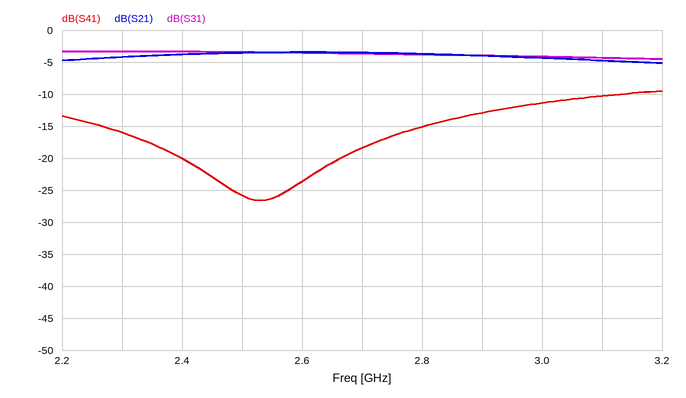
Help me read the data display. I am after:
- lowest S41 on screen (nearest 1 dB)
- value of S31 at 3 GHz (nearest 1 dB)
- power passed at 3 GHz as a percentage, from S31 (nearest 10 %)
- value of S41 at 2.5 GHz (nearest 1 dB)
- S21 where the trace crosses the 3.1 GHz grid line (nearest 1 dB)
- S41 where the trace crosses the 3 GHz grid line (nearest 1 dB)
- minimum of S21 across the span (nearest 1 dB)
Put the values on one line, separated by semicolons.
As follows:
-27 dB; -4 dB; 40 %; -26 dB; -5 dB; -11 dB; -5 dB
